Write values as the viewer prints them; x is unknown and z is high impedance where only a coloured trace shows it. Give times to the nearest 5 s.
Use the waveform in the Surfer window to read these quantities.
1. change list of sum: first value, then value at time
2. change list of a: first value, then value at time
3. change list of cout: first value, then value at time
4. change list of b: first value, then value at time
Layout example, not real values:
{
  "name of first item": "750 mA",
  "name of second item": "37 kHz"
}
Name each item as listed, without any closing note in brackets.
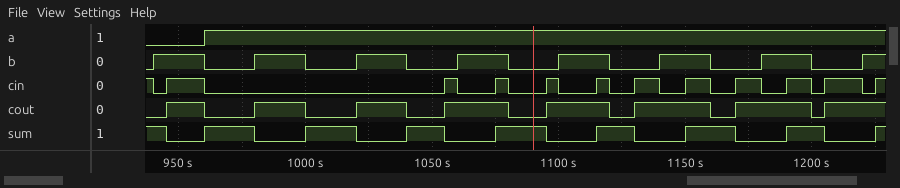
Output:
{
  "change list of sum: first value, then value at time": "1, 0 at 945 s, 1 at 960 s, 0 at 980 s, 1 at 1000 s, 0 at 1020 s, 1 at 1040 s, 0 at 1055 s, 1 at 1075 s, 0 at 1095 s, 1 at 1115 s, 0 at 1130 s, 1 at 1150 s, 0 at 1170 s, 1 at 1190 s, 0 at 1205 s, 1 at 1225 s",
  "change list of a: first value, then value at time": "0, 1 at 960 s",
  "change list of cout: first value, then value at time": "0, 1 at 945 s, 0 at 960 s, 1 at 980 s, 0 at 1000 s, 1 at 1020 s, 0 at 1040 s, 1 at 1055 s, 0 at 1080 s, 1 at 1095 s, 0 at 1120 s, 1 at 1130 s, 0 at 1160 s, 1 at 1170 s, 0 at 1200 s, 1 at 1205 s",
  "change list of b: first value, then value at time": "0, 1 at 940 s, 0 at 960 s, 1 at 980 s, 0 at 1000 s, 1 at 1020 s, 0 at 1040 s, 1 at 1060 s, 0 at 1080 s, 1 at 1100 s, 0 at 1120 s, 1 at 1140 s, 0 at 1160 s, 1 at 1180 s, 0 at 1200 s, 1 at 1220 s"
}
